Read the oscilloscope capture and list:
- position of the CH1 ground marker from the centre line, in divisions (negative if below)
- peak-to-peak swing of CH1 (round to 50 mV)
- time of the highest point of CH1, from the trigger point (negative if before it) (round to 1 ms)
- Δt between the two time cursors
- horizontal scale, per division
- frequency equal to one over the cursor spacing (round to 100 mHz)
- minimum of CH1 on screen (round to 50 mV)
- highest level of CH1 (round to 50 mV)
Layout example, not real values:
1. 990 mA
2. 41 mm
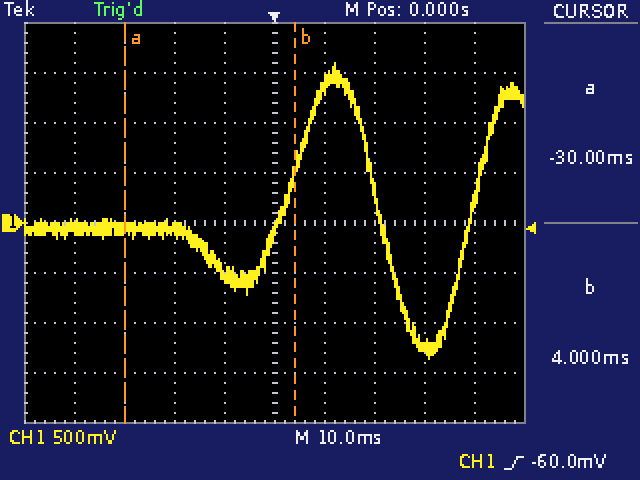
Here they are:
1. 0.0 div
2. 2.95 V
3. +12 ms
4. 34 ms
5. 10 ms
6. 29.4 Hz
7. -1.35 V
8. 1.60 V
